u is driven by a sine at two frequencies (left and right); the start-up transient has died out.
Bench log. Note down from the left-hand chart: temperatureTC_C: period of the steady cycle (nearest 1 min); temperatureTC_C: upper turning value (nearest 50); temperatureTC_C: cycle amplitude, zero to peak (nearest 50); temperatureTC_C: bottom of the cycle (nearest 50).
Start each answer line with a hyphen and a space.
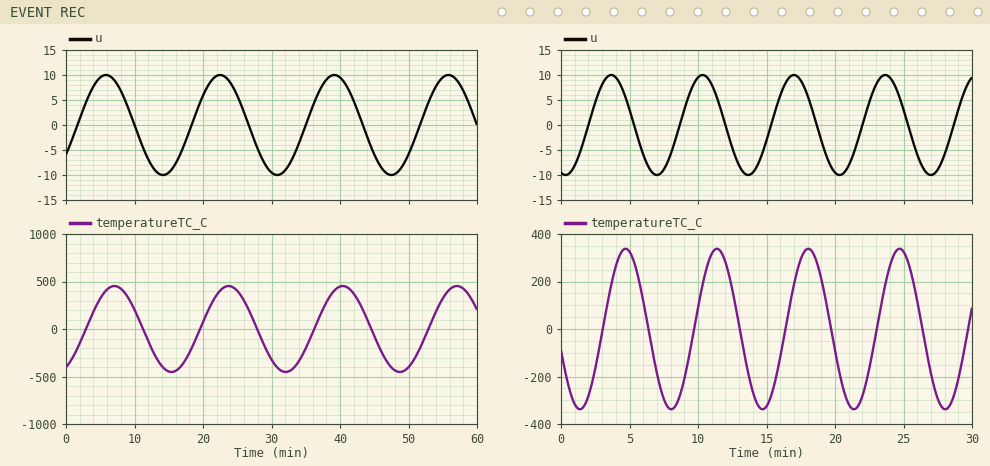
- 17 min
- 450
- 450
- -450
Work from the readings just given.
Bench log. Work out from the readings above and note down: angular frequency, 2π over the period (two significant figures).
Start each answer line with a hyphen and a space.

- 0.37 rad/min
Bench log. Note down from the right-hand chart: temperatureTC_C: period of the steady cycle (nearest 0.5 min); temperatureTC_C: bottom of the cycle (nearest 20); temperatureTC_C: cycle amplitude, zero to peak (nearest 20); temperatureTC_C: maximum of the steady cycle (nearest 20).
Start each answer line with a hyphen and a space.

- 6.5 min
- -340
- 340
- 340
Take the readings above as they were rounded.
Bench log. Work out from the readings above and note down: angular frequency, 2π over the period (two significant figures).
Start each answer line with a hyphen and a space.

- 0.97 rad/min
